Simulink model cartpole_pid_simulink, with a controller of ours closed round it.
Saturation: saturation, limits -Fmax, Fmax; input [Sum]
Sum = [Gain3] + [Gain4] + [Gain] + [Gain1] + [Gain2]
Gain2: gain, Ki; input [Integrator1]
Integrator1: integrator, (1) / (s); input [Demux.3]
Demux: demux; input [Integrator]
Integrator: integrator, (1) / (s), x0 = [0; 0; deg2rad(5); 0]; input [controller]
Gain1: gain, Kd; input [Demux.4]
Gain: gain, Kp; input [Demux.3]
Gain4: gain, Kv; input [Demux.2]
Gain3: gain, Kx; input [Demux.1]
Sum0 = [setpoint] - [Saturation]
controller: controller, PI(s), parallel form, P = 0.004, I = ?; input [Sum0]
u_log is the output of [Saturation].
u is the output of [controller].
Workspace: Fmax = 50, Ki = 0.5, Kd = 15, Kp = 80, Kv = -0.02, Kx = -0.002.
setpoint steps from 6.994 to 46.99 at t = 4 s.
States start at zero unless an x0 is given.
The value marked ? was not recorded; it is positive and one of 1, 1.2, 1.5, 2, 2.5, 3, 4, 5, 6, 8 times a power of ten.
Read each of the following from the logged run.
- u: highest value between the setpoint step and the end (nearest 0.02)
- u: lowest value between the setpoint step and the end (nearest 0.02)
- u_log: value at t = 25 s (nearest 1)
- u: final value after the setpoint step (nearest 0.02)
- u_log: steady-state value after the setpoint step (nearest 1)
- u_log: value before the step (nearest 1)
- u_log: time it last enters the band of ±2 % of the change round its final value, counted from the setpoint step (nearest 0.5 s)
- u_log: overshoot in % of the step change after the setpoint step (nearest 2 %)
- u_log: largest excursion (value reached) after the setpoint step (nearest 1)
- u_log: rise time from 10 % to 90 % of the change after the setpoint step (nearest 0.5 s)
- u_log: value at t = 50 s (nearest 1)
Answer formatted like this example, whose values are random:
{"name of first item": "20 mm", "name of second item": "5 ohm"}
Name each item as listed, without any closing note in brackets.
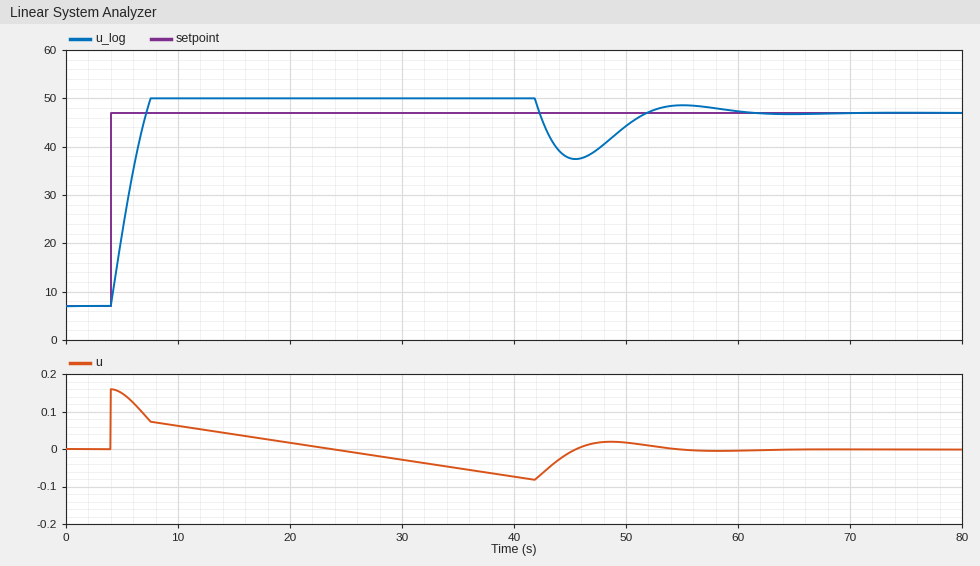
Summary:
{"u: highest value between the setpoint step and the end": "0.16", "u: lowest value between the setpoint step and the end": "-0.08", "u_log: value at t = 25 s": "50", "u: final value after the setpoint step": "0.00", "u_log: steady-state value after the setpoint step": "47", "u_log: value before the step": "7", "u_log: time it last enters the band of ±2 % of the change round its final value, counted from the setpoint step": "54.5 s", "u_log: overshoot in % of the step change after the setpoint step": "8 %", "u_log: largest excursion (value reached) after the setpoint step": "50", "u_log: rise time from 10 % to 90 % of the change after the setpoint step": "2.5 s", "u_log: value at t = 50 s": "44"}
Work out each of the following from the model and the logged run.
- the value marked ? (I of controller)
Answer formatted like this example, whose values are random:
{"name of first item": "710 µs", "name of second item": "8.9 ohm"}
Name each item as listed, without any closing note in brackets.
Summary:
{"the value marked ?": "0.0015"}
